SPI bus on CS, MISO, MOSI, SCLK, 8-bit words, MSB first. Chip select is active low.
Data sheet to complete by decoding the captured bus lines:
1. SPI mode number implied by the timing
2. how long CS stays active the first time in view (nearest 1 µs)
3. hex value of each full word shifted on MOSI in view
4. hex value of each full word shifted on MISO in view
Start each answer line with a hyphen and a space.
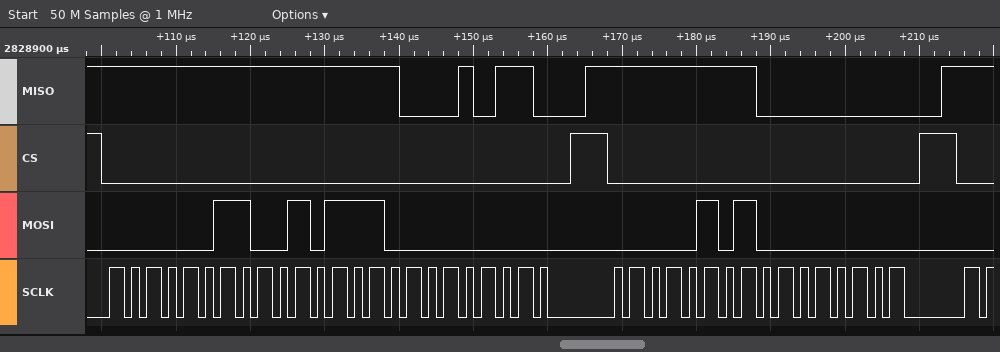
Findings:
- 0
- 63 µs
- 03, 2E, 00, 05, 00
- FF, FF, 16, FF, 00
